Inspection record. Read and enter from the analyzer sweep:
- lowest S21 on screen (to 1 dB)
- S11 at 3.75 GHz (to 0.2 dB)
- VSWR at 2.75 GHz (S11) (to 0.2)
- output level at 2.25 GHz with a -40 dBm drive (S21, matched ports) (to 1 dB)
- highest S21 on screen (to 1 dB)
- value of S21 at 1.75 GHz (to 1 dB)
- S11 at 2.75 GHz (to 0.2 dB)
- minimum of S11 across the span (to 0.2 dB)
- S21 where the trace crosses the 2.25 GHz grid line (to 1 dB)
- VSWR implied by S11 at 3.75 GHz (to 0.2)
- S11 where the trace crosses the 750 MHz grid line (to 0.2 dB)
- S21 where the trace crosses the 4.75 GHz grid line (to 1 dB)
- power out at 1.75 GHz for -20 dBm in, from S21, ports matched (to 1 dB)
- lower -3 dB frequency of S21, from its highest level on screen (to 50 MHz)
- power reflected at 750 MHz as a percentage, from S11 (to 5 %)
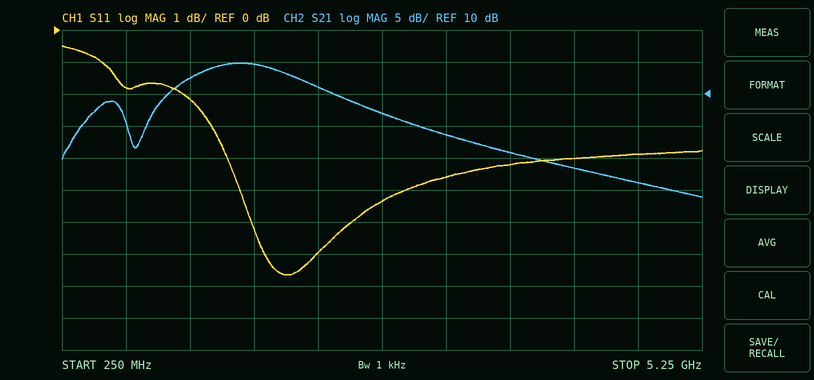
-6 dB
-4.2 dB
3.4
-29 dBm
15 dB
15 dB
-5.4 dB
-7.6 dB
11 dB
4.2
-1.8 dB
-4 dB
-5 dBm
1.20 GHz
65 %
